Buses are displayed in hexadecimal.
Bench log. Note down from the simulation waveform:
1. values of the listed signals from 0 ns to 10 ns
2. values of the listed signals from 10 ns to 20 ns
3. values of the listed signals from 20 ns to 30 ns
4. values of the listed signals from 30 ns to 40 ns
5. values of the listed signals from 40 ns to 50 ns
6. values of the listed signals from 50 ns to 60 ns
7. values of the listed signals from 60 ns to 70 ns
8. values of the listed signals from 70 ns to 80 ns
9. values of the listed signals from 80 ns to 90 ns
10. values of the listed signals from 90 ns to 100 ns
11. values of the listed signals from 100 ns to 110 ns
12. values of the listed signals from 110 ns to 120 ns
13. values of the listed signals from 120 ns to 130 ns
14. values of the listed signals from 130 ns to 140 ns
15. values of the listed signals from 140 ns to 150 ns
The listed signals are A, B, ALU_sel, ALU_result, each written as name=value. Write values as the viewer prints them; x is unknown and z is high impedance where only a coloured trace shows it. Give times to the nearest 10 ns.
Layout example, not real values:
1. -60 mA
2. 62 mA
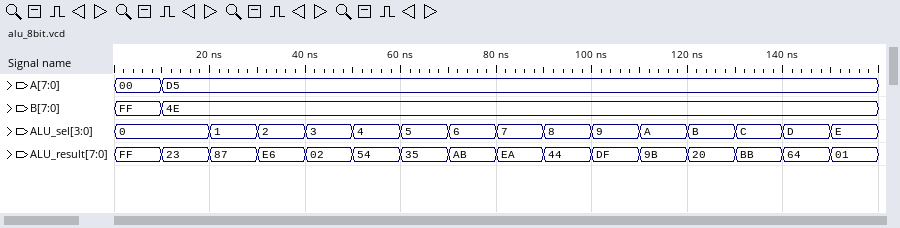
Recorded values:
1. A=00, B=FF, ALU_sel=0, ALU_result=FF
2. A=D5, B=4E, ALU_sel=0, ALU_result=23
3. A=D5, B=4E, ALU_sel=1, ALU_result=87
4. A=D5, B=4E, ALU_sel=2, ALU_result=E6
5. A=D5, B=4E, ALU_sel=3, ALU_result=02
6. A=D5, B=4E, ALU_sel=4, ALU_result=54
7. A=D5, B=4E, ALU_sel=5, ALU_result=35
8. A=D5, B=4E, ALU_sel=6, ALU_result=AB
9. A=D5, B=4E, ALU_sel=7, ALU_result=EA
10. A=D5, B=4E, ALU_sel=8, ALU_result=44
11. A=D5, B=4E, ALU_sel=9, ALU_result=DF
12. A=D5, B=4E, ALU_sel=A, ALU_result=9B
13. A=D5, B=4E, ALU_sel=B, ALU_result=20
14. A=D5, B=4E, ALU_sel=C, ALU_result=BB
15. A=D5, B=4E, ALU_sel=D, ALU_result=64
